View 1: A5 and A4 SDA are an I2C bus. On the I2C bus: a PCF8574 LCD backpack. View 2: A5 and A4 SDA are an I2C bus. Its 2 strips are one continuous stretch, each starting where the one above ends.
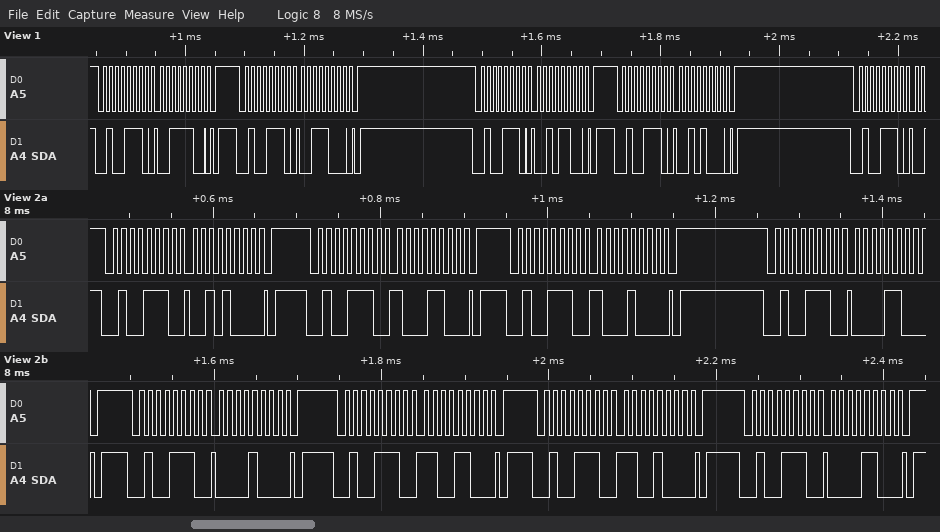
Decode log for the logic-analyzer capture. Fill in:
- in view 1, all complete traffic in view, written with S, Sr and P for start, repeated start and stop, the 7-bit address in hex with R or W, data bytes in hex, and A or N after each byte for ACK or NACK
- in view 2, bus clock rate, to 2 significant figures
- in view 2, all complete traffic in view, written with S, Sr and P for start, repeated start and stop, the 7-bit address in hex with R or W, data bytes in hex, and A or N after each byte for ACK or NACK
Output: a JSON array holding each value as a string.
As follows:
["S 27W A 3C A P S 27W A 38 A P S 27W A 2C A P S 27W A 28 A P S 27W A", "100 kHz", "S 27W A 28 A P S 27W A 8C A P S 27W A 88 A P S 27W A 0C A P S 27W A 08 A P S 27W A CC A P S 27W A C8 A P S 27W A 0C A P"]
